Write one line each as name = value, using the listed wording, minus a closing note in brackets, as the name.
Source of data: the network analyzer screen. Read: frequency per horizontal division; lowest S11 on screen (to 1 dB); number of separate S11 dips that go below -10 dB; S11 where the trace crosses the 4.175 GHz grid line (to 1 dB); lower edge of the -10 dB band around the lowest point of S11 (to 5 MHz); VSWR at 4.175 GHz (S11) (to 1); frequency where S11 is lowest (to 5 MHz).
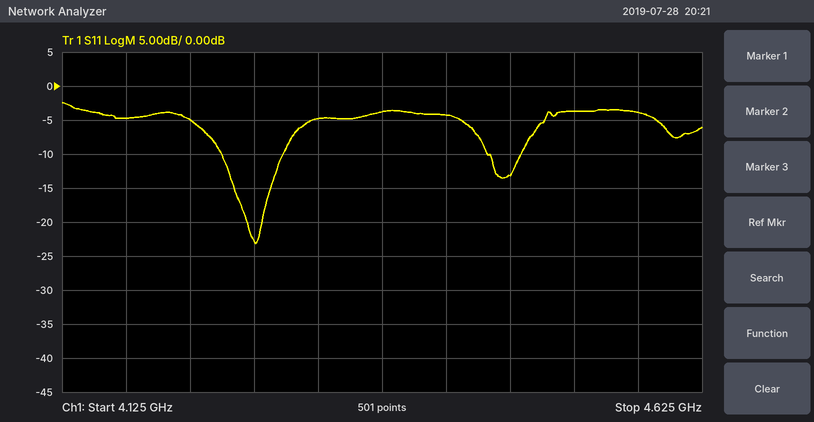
frequency per horizontal division = 50 MHz
lowest S11 on screen = -23 dB
number of separate S11 dips that go below -10 dB = 2
S11 where the trace crosses the 4.175 GHz grid line = -5 dB
lower edge of the -10 dB band around the lowest point of S11 = 4.250 GHz
VSWR at 4.175 GHz (S11) = 4
frequency where S11 is lowest = 4.275 GHz
